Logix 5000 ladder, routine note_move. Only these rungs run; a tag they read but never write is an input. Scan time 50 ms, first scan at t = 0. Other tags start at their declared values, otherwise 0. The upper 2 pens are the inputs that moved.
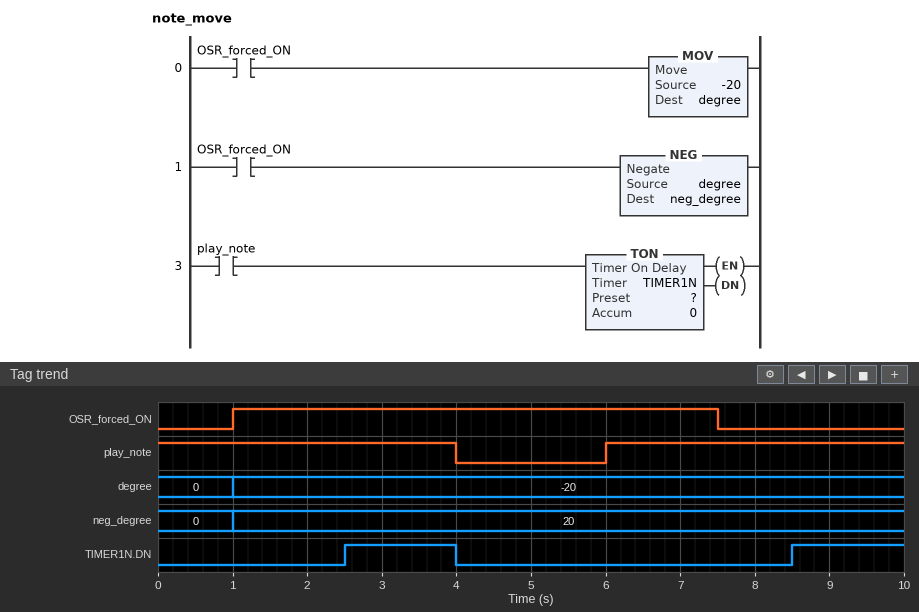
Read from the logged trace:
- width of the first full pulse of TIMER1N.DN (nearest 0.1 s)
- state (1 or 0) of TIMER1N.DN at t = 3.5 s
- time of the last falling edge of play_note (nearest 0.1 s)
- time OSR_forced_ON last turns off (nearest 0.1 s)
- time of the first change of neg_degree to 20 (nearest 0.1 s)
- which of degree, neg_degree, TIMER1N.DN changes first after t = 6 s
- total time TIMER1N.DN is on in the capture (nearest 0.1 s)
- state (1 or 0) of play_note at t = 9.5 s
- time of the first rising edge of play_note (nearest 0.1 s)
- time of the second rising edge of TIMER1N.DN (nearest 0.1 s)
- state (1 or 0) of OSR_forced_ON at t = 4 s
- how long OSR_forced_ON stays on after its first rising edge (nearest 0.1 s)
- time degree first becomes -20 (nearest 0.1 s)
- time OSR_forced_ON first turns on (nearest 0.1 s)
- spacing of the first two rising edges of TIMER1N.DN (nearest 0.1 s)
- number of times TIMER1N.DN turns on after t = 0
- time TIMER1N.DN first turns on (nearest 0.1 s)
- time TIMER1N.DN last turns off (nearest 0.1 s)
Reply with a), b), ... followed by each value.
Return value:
a) 1.5 s
b) 1
c) 4.0 s
d) 7.5 s
e) 1.0 s
f) TIMER1N.DN
g) 3.0 s
h) 1
i) 6.0 s
j) 8.5 s
k) 1
l) 6.5 s
m) 1.0 s
n) 1.0 s
o) 6.0 s
p) 2
q) 2.5 s
r) 4.0 s
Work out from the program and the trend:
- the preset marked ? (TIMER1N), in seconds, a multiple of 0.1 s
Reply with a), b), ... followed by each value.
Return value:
a) 2.5 s
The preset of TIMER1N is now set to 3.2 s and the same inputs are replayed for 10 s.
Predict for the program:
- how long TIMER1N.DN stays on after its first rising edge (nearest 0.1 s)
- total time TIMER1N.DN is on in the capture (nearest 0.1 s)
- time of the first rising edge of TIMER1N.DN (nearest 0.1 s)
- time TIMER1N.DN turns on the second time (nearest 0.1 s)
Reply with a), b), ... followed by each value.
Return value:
a) 0.8 s
b) 1.6 s
c) 3.2 s
d) 9.2 s
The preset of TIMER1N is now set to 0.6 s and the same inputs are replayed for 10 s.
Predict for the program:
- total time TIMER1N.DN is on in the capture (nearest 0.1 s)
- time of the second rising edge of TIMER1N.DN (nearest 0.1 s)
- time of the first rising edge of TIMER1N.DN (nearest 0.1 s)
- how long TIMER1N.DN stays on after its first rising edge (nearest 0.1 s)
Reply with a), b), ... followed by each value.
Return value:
a) 6.8 s
b) 6.6 s
c) 0.6 s
d) 3.4 s
